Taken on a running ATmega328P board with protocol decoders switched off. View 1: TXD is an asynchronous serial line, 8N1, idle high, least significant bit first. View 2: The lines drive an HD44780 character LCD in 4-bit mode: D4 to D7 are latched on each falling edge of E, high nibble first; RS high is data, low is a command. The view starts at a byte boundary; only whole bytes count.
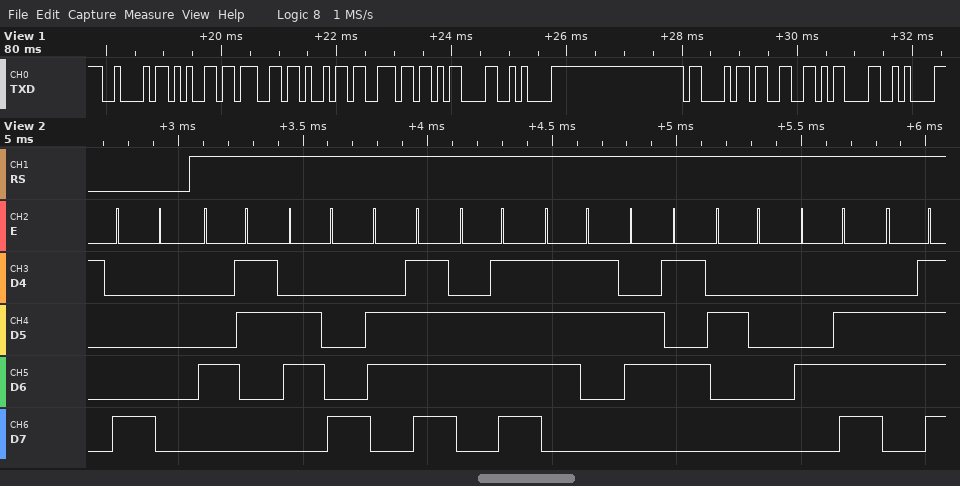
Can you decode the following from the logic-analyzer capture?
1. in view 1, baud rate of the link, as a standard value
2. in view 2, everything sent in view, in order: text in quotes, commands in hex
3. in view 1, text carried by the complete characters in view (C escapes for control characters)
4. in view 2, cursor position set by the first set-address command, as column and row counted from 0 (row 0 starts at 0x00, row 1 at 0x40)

9600 baud
0x80 "Choose No"
"Begin\r\nC3\r\n"
column 0, row 0
